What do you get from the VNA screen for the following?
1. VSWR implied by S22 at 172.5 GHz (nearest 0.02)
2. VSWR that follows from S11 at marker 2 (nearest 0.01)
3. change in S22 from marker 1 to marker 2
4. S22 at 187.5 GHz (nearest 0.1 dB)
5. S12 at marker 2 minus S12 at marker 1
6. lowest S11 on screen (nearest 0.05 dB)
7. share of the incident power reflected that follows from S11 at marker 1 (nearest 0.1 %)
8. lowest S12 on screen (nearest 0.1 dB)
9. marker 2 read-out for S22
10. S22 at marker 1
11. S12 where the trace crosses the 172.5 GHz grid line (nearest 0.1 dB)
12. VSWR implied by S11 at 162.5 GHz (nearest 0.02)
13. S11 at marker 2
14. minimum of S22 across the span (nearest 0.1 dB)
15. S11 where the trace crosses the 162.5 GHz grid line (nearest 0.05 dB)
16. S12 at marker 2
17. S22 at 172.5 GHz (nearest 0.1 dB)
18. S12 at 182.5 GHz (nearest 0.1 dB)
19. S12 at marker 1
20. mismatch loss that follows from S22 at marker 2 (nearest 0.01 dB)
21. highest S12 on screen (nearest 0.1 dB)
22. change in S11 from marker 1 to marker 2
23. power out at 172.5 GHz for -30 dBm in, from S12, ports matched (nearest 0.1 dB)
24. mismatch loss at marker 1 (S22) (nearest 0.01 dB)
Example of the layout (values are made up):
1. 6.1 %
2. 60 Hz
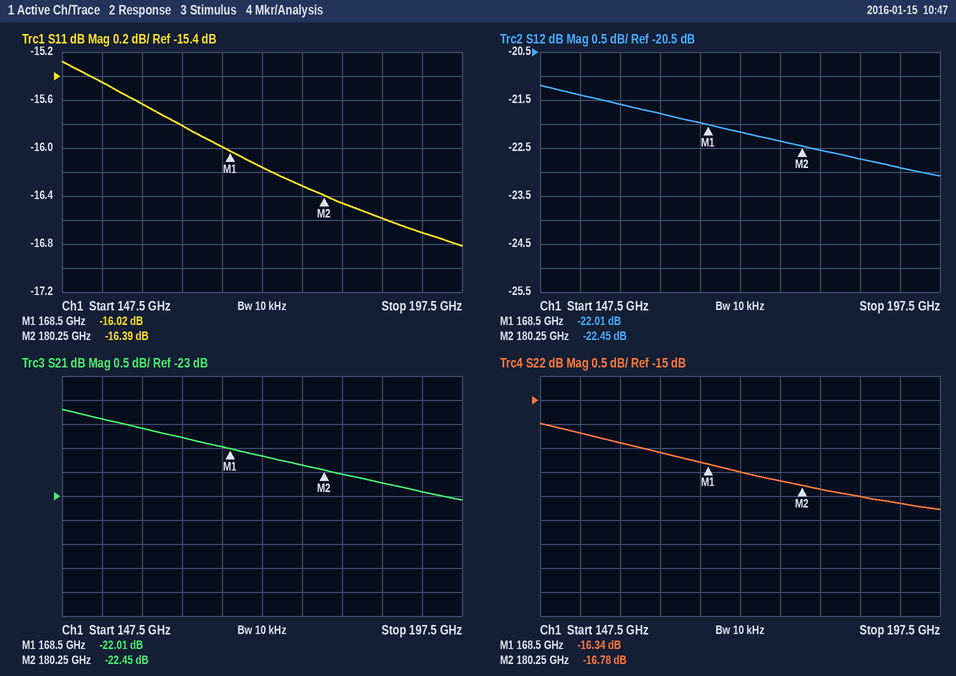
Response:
1. 1.36
2. 1.36
3. -0.44 dB
4. -17.0 dB
5. -0.44 dB
6. -16.80 dB
7. 2.5 %
8. -23.1 dB
9. -16.78 dB
10. -16.34 dB
11. -22.2 dB
12. 1.38
13. -16.39 dB
14. -17.3 dB
15. -15.80 dB
16. -22.45 dB
17. -16.5 dB
18. -22.5 dB
19. -22.01 dB
20. 0.09 dB
21. -21.2 dB
22. -0.37 dB
23. -52.2 dBm
24. 0.10 dB
